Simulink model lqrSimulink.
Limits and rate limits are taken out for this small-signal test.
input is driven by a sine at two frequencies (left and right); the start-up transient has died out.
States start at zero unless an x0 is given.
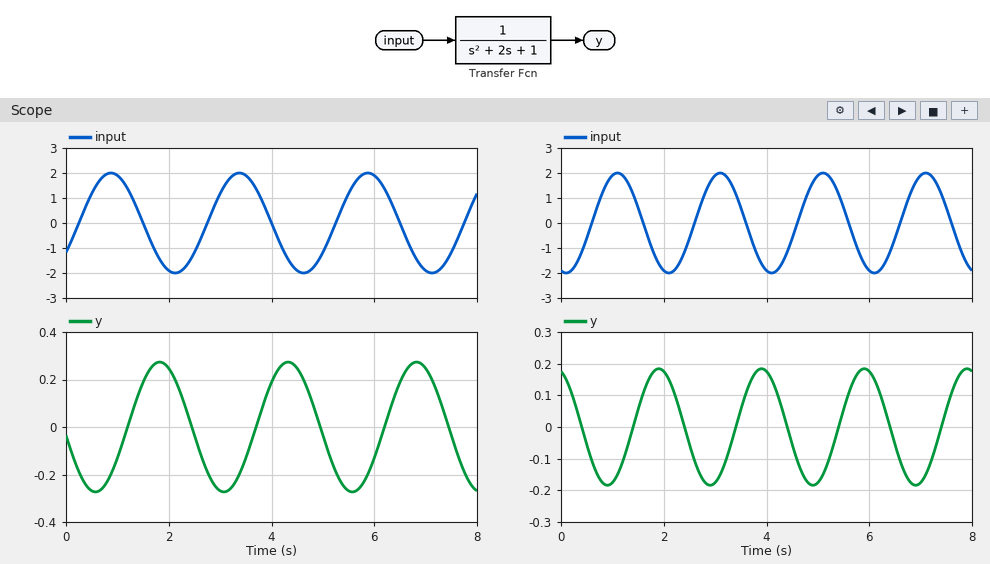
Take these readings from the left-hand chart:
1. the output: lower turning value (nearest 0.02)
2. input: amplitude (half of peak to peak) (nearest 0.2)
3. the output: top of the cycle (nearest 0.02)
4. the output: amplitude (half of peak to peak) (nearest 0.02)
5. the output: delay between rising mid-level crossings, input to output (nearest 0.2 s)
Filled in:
-0.28
2.0
0.28
0.28
1.0 s
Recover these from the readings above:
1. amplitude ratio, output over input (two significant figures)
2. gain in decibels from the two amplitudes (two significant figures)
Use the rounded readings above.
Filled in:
0.14
-17 dB
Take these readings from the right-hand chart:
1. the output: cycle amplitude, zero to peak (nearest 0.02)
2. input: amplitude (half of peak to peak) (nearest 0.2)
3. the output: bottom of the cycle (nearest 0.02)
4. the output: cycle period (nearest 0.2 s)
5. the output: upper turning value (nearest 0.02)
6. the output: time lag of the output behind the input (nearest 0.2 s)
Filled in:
0.18
2.0
-0.18
2.0 s
0.18
0.8 s
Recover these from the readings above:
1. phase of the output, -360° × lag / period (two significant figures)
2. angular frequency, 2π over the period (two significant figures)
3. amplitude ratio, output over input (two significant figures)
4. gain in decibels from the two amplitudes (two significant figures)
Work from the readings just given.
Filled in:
-140°
3.1 rad/s
0.090
-21 dB
